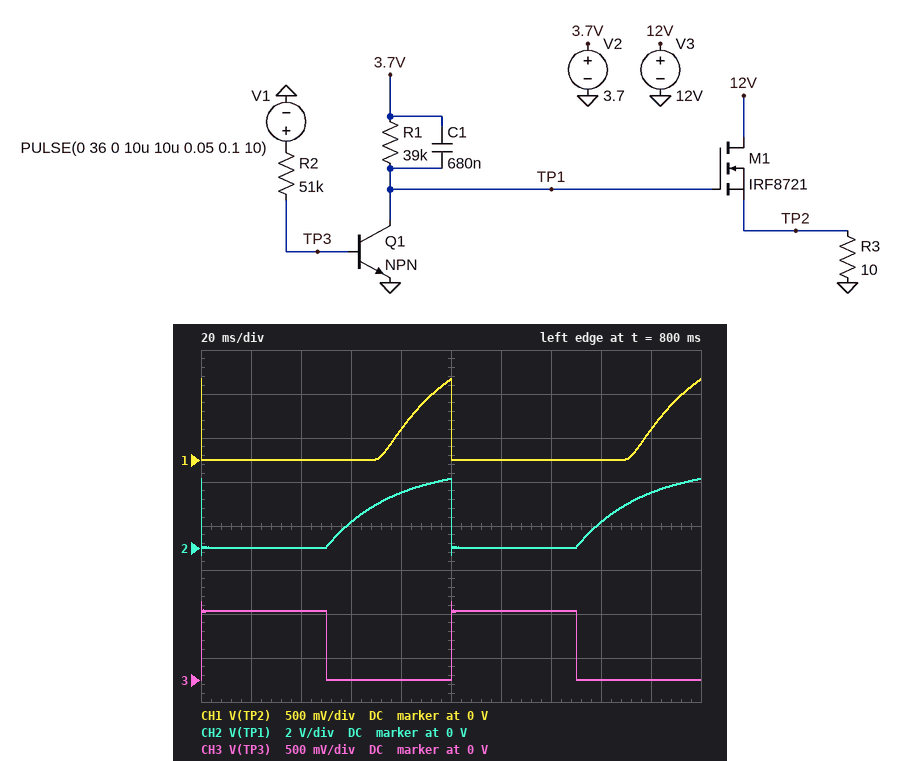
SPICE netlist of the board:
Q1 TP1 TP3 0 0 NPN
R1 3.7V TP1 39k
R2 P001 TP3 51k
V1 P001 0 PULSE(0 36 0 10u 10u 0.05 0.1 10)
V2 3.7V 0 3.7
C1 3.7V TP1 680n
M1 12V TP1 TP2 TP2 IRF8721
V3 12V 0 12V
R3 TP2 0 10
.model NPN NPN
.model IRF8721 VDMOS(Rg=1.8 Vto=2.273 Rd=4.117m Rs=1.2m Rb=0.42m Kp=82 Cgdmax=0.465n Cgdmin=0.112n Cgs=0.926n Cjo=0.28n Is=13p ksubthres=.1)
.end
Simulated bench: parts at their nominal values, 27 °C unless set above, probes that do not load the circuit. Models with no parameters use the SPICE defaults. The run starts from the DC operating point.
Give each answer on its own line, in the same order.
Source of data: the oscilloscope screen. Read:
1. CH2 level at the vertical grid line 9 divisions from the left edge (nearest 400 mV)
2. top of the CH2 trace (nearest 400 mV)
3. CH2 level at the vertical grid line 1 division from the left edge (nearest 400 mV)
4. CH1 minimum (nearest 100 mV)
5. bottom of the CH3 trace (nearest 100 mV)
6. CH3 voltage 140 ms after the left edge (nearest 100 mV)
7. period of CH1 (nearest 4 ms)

2.4 V
3.2 V
0 V
0 V
0 V
800 mV
100 ms
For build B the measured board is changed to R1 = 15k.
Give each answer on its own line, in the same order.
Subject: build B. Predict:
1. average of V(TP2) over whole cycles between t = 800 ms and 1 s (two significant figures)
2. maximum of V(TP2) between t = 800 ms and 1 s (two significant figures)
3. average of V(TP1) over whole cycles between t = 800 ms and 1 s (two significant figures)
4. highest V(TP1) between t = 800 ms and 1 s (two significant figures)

450 mV
1.4 V
1.5 V
3.7 V
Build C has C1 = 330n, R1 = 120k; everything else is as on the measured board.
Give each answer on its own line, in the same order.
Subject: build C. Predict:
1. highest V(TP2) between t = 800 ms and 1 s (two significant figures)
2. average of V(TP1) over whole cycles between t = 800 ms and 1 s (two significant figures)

470 mV
810 mV
